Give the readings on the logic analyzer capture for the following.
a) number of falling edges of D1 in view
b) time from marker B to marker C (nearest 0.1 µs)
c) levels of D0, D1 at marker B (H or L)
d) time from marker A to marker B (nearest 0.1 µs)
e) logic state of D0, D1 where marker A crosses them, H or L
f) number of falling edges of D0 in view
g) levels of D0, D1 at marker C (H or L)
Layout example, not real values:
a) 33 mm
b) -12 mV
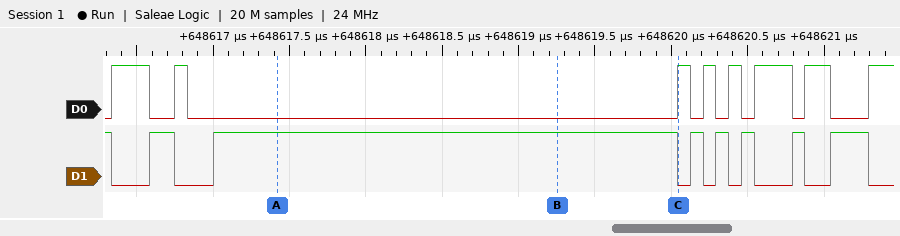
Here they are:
a) 8
b) 0.8 µs
c) D0=L, D1=H
d) 1.8 µs
e) D0=L, D1=H
f) 7
g) D0=H, D1=L
